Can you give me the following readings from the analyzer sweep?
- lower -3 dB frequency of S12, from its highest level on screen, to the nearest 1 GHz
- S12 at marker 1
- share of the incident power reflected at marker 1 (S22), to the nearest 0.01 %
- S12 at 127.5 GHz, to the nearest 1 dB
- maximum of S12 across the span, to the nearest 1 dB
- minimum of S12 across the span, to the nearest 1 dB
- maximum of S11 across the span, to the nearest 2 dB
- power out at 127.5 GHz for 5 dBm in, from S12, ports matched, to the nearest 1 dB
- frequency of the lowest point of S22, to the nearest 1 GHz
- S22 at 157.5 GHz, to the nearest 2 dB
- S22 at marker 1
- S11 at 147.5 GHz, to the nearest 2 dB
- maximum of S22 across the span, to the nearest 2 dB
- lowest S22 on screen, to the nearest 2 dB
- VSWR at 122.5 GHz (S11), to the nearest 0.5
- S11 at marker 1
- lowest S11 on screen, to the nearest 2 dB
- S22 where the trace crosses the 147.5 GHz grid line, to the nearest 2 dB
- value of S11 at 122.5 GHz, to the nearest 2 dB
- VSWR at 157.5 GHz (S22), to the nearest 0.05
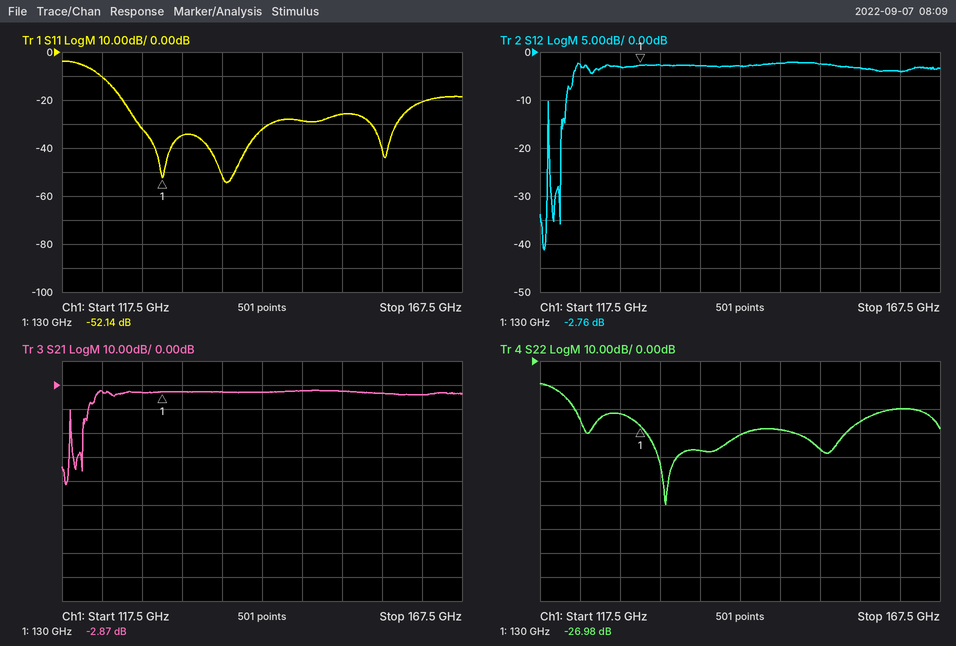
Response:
122 GHz
-2.76 dB
0.20 %
-3 dB
-2 dB
-41 dB
-4 dB
2 dBm
133 GHz
-26 dB
-26.98 dB
-28 dB
-10 dB
-60 dB
2.0
-52.14 dB
-54 dB
-28 dB
-10 dB
1.10
